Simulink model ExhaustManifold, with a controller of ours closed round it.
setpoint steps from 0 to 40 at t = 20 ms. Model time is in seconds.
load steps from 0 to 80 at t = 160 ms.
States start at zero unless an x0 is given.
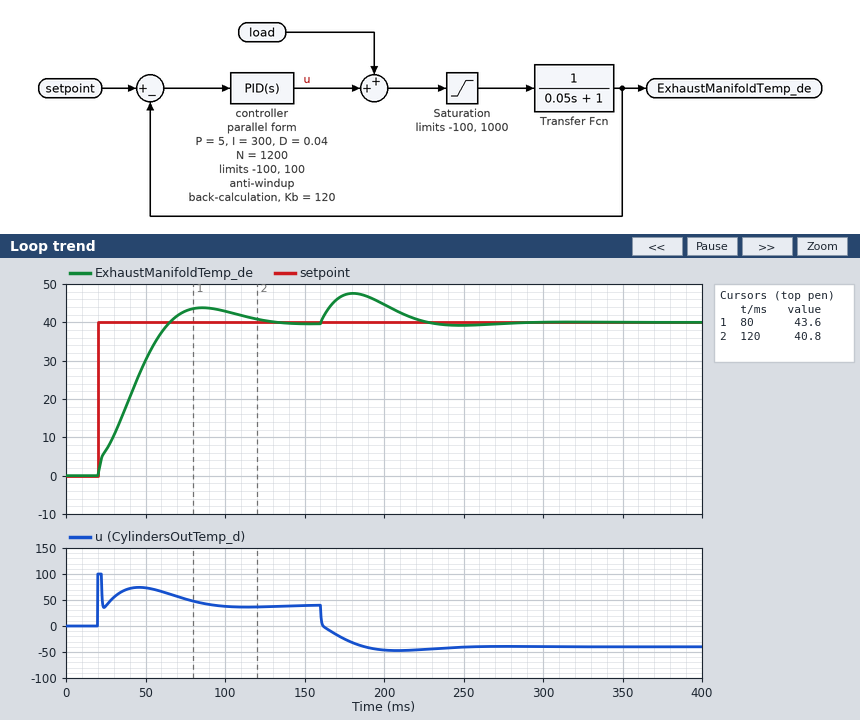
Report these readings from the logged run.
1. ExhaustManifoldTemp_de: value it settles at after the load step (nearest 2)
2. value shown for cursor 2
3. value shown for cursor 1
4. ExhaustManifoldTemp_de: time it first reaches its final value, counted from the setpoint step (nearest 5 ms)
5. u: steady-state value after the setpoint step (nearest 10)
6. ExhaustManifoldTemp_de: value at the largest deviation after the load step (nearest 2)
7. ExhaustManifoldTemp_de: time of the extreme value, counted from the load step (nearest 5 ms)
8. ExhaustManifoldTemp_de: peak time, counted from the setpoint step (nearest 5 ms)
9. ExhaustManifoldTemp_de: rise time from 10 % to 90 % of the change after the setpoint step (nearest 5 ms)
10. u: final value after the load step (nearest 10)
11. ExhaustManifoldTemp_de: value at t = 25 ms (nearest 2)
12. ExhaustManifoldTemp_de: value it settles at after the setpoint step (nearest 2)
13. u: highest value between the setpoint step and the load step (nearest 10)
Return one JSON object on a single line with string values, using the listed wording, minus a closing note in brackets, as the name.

{"ExhaustManifoldTemp_de: value it settles at after the load step": "40", "value shown for cursor 2": "40.8", "value shown for cursor 1": "43.6", "ExhaustManifoldTemp_de: time it first reaches its final value, counted from the setpoint step": "45 ms", "u: steady-state value after the setpoint step": "40", "ExhaustManifoldTemp_de: value at the largest deviation after the load step": "48", "ExhaustManifoldTemp_de: time of the extreme value, counted from the load step": "20 ms", "ExhaustManifoldTemp_de: peak time, counted from the setpoint step": "65 ms", "ExhaustManifoldTemp_de: rise time from 10 % to 90 % of the change after the setpoint step": "35 ms", "u: final value after the load step": "-40", "ExhaustManifoldTemp_de: value at t = 25 ms": "6", "ExhaustManifoldTemp_de: value it settles at after the setpoint step": "40", "u: highest value between the setpoint step and the load step": "100"}
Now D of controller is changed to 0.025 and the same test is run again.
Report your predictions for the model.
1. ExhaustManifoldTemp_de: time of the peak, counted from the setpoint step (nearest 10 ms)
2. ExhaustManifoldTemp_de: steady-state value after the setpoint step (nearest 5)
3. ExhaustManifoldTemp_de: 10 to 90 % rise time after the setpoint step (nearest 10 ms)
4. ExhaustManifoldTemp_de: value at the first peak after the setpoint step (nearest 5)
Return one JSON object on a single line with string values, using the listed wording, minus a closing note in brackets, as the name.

{"ExhaustManifoldTemp_de: time of the peak, counted from the setpoint step": "60 ms", "ExhaustManifoldTemp_de: steady-state value after the setpoint step": "40", "ExhaustManifoldTemp_de: 10 to 90 % rise time after the setpoint step": "30 ms", "ExhaustManifoldTemp_de: value at the first peak after the setpoint step": "45"}
